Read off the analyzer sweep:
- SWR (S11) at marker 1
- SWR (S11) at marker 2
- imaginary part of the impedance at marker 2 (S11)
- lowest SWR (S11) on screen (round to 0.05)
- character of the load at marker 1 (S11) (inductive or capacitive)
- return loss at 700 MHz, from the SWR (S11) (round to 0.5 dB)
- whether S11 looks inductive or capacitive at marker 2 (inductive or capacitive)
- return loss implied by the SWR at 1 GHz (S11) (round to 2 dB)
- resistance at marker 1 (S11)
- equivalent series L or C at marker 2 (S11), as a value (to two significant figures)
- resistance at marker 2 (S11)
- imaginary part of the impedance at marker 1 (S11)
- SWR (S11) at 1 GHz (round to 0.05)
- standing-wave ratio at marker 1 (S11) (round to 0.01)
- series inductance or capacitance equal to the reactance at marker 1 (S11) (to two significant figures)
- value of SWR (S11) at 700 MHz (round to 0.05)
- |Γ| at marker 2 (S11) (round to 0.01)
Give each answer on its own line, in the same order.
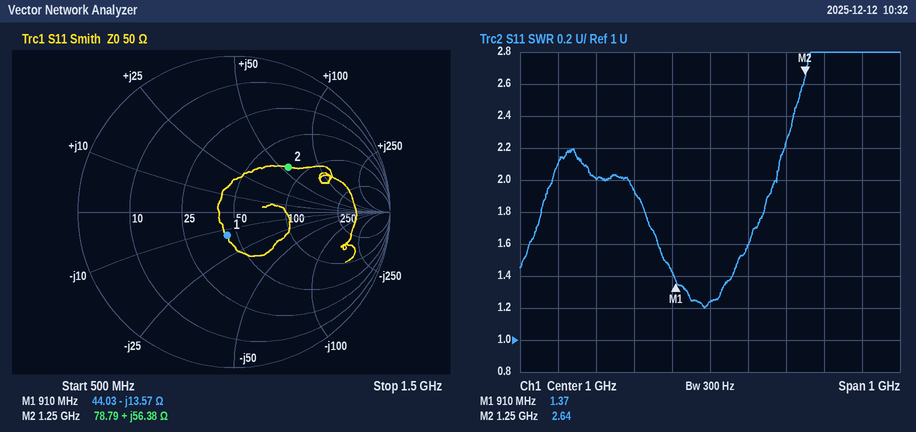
1.37
2.64
+56.38 Ω
1.20
capacitive
9.5 dB
inductive
20 dB
44.03 Ω
7.2 nH
78.79 Ω
-13.57 Ω
1.25
1.37
13 pF
2.00
0.45
